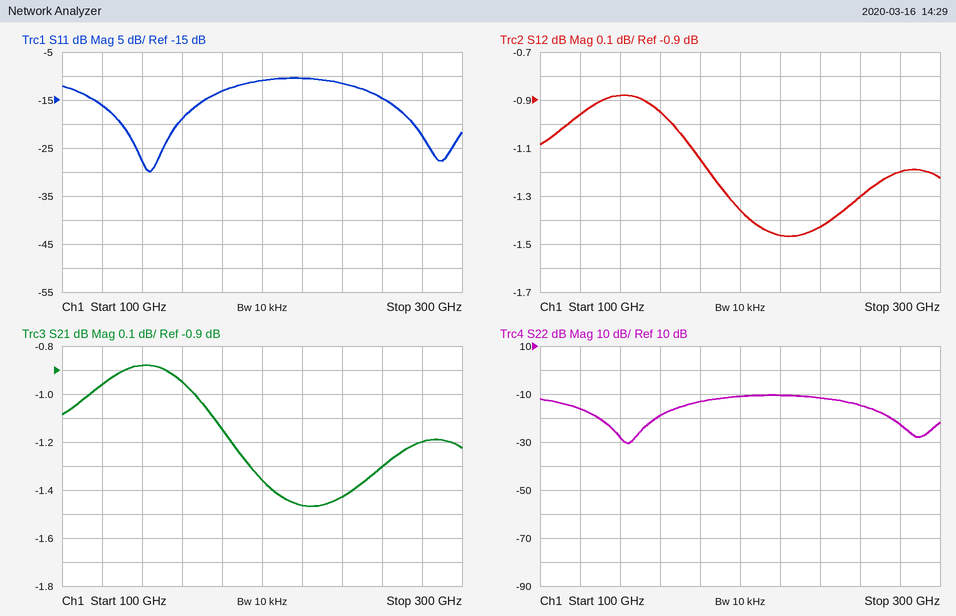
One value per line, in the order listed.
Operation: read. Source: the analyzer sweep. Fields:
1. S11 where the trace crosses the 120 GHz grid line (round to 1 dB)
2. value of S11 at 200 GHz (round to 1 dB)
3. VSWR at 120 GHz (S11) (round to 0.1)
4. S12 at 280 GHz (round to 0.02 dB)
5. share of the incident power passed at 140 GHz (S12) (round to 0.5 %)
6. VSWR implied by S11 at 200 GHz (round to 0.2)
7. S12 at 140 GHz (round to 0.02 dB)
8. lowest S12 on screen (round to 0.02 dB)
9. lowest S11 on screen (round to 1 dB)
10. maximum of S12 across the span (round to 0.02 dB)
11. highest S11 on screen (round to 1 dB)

-16 dB
-11 dB
1.4
-1.20 dB
81.5 %
1.8
-0.88 dB
-1.46 dB
-30 dB
-0.88 dB
-10 dB
